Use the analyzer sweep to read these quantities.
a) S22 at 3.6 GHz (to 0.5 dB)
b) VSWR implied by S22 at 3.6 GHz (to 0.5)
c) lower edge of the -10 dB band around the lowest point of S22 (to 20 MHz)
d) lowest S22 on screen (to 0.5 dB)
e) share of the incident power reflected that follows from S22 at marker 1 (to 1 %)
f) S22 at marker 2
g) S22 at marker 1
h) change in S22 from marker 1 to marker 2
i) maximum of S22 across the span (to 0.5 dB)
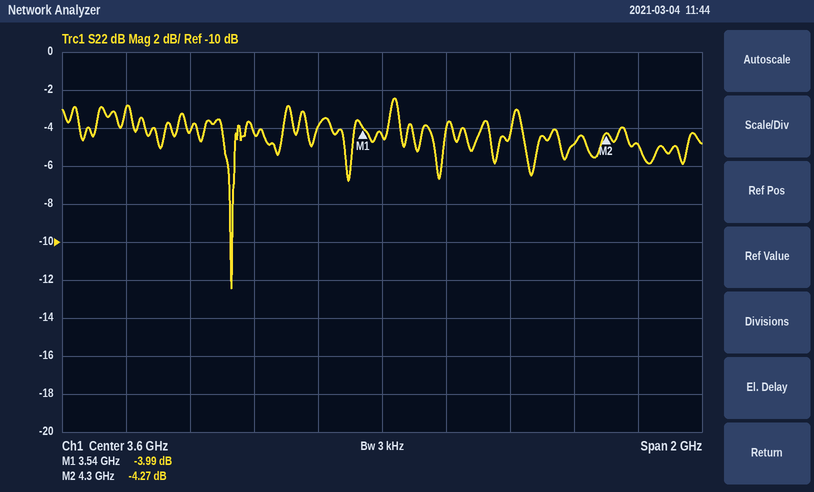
-4.5 dB
4.0
3.12 GHz
-12.5 dB
40 %
-4.27 dB
-3.99 dB
-0.28 dB
-2.5 dB
